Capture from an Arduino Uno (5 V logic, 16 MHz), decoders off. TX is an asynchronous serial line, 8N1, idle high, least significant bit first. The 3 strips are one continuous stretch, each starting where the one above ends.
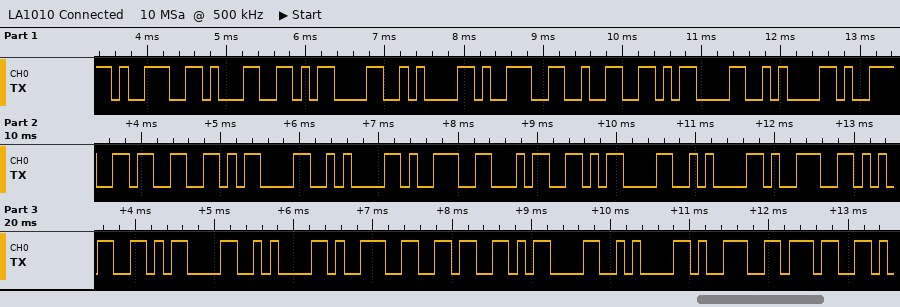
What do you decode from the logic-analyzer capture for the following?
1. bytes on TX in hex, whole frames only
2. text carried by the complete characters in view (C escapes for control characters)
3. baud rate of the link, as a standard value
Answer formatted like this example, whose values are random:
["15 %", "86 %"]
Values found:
["39 31 0D 0A 39 32 0D 0A 39 33 0D 0A 39 34 0D 0A 39 35 0D 0A 39 36 0D 0A 39 37", "\"91\\r\\n92\\r\\n93\\r\\n94\\r\\n95\\r\\n96\\r\\n97\"", "9600 baud"]
